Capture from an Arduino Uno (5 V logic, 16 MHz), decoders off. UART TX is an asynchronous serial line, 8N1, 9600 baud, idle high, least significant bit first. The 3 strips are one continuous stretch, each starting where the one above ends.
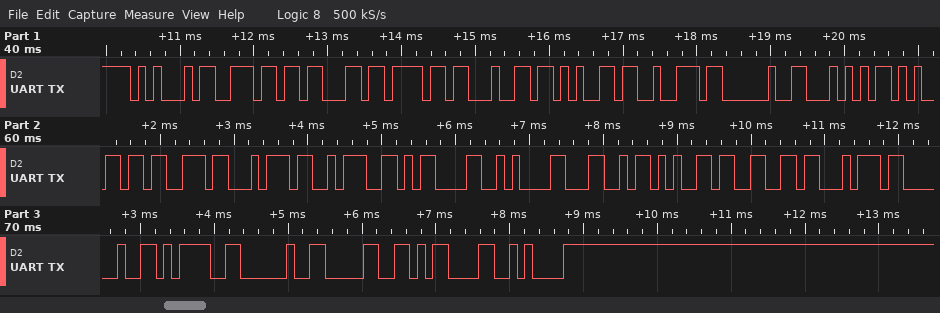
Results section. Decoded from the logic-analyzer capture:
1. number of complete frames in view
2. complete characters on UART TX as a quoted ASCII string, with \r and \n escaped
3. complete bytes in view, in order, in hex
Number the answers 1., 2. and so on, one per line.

1. 25
2. "Encoder Test:\r\nLeft = 0\r\n"
3. 45 6E 63 6F 64 65 72 20 54 65 73 74 3A 0D 0A 4C 65 66 74 20 3D 20 30 0D 0A
